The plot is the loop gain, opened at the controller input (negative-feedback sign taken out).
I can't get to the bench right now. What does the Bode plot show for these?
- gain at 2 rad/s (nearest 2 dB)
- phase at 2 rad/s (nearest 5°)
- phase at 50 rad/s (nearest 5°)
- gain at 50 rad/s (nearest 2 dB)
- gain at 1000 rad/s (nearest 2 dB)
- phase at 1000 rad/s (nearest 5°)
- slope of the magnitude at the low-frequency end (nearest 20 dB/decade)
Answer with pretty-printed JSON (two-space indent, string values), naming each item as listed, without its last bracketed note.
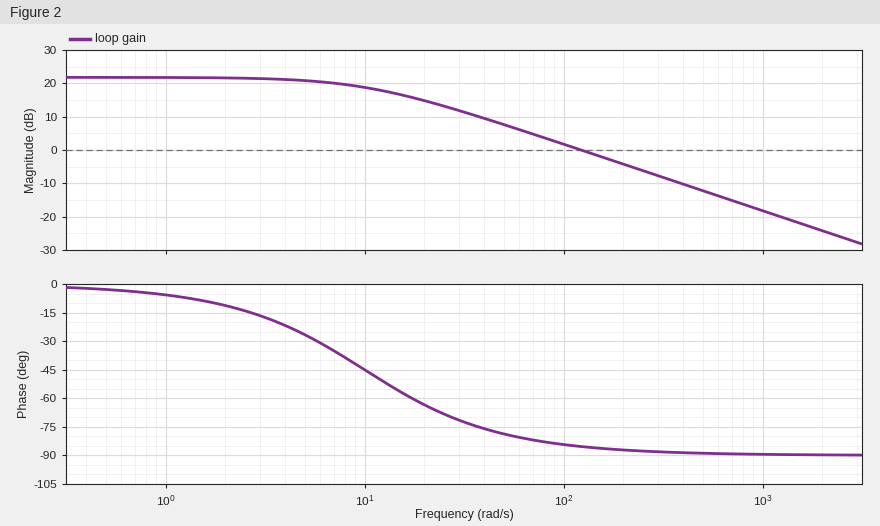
{
  "gain at 2 rad/s": "22 dB",
  "phase at 2 rad/s": "-10°",
  "phase at 50 rad/s": "-80°",
  "gain at 50 rad/s": "8 dB",
  "gain at 1000 rad/s": "-18 dB",
  "phase at 1000 rad/s": "-90°",
  "slope of the magnitude at the low-frequency end": "0 dB/decade"
}
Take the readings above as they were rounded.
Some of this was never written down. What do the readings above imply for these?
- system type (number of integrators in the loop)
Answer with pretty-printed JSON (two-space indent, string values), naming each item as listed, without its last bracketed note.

{
  "system type": "0"
}
